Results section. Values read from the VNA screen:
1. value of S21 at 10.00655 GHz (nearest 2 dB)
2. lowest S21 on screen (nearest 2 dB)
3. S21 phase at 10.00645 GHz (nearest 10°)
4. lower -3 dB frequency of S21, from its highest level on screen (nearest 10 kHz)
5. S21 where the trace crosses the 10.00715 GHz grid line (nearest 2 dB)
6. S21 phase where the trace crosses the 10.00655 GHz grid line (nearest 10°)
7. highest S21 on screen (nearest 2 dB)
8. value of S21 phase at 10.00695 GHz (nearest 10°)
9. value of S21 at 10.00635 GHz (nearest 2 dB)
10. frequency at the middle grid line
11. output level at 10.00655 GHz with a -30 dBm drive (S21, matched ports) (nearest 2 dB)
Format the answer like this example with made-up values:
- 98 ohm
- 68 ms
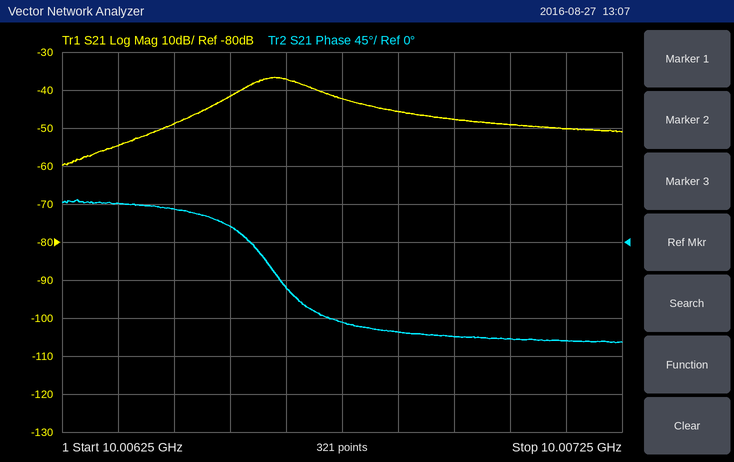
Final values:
- -42 dB
- -60 dB
- 40°
- 10.00657 GHz
- -50 dB
- 20°
- -36 dB
- -110°
- -54 dB
- 10.00675 GHz
- -72 dBm
